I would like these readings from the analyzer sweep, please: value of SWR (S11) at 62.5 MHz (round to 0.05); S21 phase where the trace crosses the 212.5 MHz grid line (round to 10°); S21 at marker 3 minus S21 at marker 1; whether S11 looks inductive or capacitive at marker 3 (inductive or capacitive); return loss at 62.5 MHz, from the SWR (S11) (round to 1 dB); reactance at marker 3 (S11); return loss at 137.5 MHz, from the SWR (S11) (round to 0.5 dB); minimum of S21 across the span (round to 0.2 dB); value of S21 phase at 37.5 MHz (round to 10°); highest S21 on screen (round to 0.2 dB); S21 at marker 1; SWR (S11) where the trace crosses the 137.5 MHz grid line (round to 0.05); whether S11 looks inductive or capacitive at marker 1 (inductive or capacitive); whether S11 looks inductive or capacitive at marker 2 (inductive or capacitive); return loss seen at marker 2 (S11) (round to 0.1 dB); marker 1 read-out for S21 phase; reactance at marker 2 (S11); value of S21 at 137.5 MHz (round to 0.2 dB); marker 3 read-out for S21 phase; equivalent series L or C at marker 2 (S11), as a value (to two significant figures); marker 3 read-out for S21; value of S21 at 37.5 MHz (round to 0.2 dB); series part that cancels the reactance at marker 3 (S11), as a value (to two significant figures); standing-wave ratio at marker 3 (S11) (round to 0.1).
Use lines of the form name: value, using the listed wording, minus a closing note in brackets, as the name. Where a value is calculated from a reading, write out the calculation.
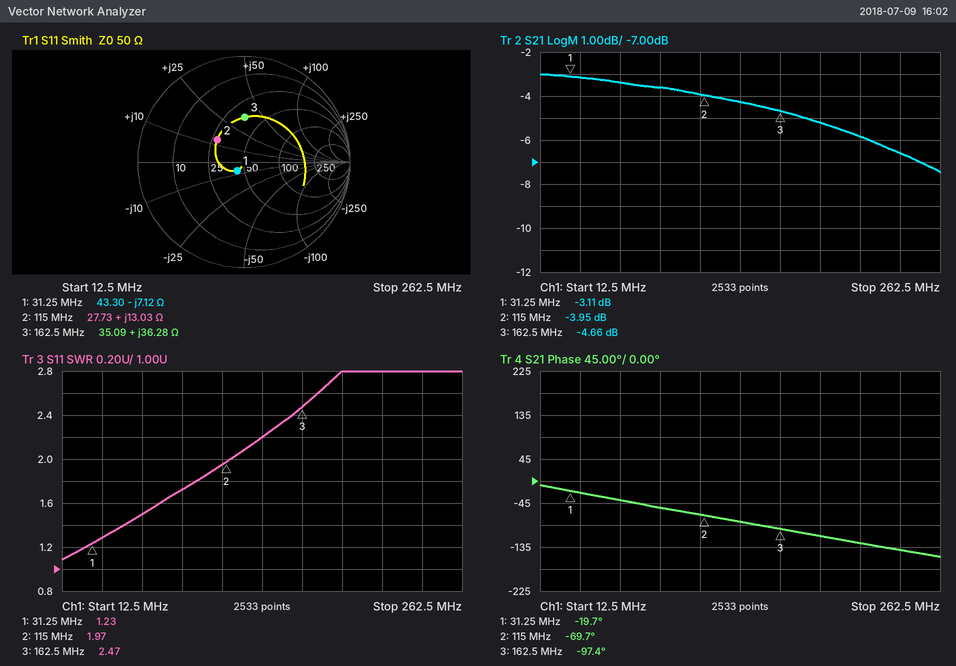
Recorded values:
value of SWR (S11) at 62.5 MHz: 1.50
S21 phase where the trace crosses the 212.5 MHz grid line: -130°
S21 at marker 3 minus S21 at marker 1: -4.66 − (-3.11) = -1.55 dB
whether S11 looks inductive or capacitive at marker 3: inductive
return loss at 62.5 MHz, from the SWR (S11): −20 log10((1.5 − 1)/(1.5 + 1)) ≈ 14 dB
reactance at marker 3: +36.28 Ω
return loss at 137.5 MHz, from the SWR (S11): −20 log10((2.2 − 1)/(2.2 + 1)) ≈ 8.5 dB
minimum of S21 across the span: -7.4 dB
value of S21 phase at 37.5 MHz: -20°
highest S21 on screen: -3.0 dB
S21 at marker 1: -3.11 dB
SWR (S11) where the trace crosses the 137.5 MHz grid line: 2.20
whether S11 looks inductive or capacitive at marker 1: capacitive
whether S11 looks inductive or capacitive at marker 2: inductive
return loss seen at marker 2 (S11): 9.7 dB
marker 1 read-out for S21 phase: -19.7°
reactance at marker 2: +13.03 Ω
value of S21 at 137.5 MHz: -4.2 dB
marker 3 read-out for S21 phase: -97.4°
equivalent series L or C at marker 2 (S11), as a value: L = 13.03 Ω/(2π × 115 MHz) ≈ 18 nH
marker 3 read-out for S21: -4.66 dB
value of S21 at 37.5 MHz: -3.2 dB
series part that cancels the reactance at marker 3 (S11), as a value: C = 1/(2π × 162.5 MHz × 36.28 Ω) ≈ 27 pF
standing-wave ratio at marker 3 (S11): 2.5
